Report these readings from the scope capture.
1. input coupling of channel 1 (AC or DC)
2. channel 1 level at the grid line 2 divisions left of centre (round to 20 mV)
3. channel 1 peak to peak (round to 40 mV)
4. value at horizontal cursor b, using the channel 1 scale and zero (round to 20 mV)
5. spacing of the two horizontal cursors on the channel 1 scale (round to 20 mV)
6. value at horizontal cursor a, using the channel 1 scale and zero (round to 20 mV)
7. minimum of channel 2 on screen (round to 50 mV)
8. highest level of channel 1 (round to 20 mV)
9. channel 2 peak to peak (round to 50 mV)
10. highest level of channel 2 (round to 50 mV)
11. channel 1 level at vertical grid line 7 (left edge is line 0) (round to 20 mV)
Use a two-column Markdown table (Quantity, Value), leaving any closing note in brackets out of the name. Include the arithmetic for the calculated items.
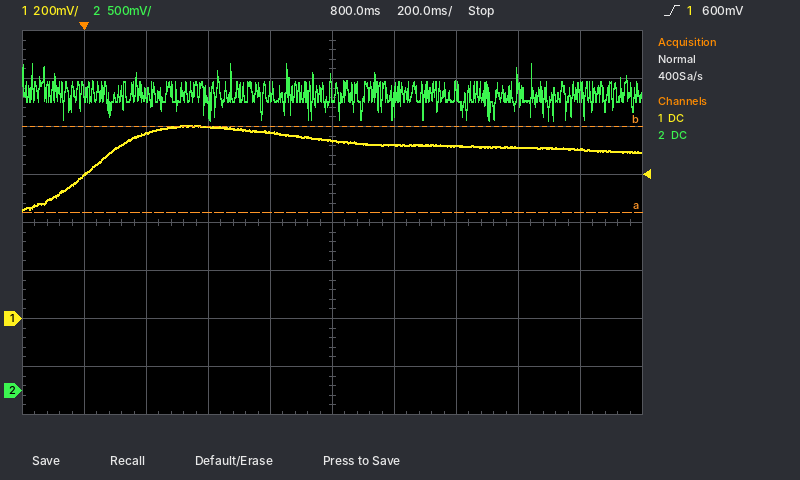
| Quantity | Value |
|---|---|
| input coupling of channel 1 | DC |
| channel 1 level at the grid line 2 divisions left of centre | 800 mV |
| channel 1 peak to peak | 360 mV |
| value at horizontal cursor b, using the channel 1 scale and zero | 800 mV |
| spacing of the two horizontal cursors on the channel 1 scale | 360 mV |
| value at horizontal cursor a, using the channel 1 scale and zero | 440 mV |
| minimum of channel 2 on screen | 2.80 V |
| highest level of channel 1 | 800 mV |
| channel 2 peak to peak | 3.40 V − (2.80 V) = 600 mV |
| highest level of channel 2 | 3.40 V |
| channel 1 level at vertical grid line 7 (left edge is line 0) | 720 mV |
